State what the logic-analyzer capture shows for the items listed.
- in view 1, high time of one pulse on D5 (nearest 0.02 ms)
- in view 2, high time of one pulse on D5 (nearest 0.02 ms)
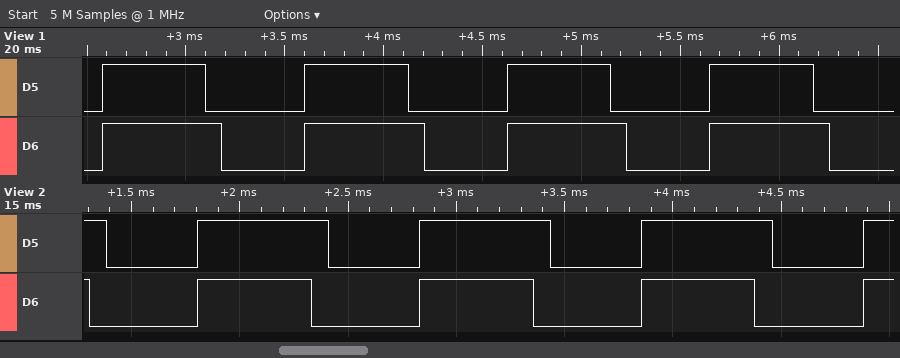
0.52 ms
0.60 ms
